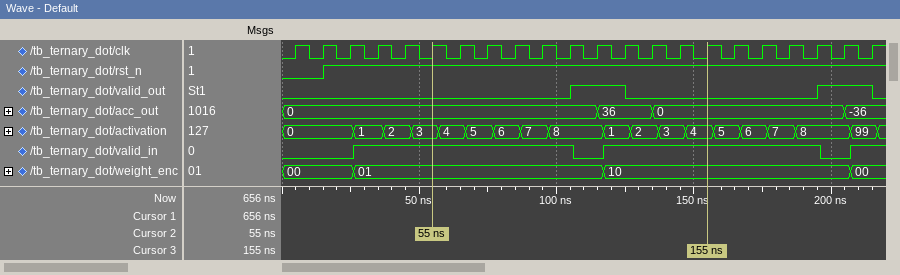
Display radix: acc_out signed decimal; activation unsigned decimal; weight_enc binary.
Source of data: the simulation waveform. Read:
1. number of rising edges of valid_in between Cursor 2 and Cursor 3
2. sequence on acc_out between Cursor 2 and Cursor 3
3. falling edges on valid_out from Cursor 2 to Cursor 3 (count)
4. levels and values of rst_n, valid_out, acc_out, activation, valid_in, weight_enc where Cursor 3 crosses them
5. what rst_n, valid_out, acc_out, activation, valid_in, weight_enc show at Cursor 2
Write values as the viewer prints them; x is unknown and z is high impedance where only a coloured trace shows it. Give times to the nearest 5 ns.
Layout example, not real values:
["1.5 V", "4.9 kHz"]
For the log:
["1", "0, 36, 0", "1", "rst_n=1, valid_out=0, acc_out=0, activation=4, valid_in=1, weight_enc=10", "rst_n=1, valid_out=0, acc_out=0, activation=3, valid_in=1, weight_enc=01"]
